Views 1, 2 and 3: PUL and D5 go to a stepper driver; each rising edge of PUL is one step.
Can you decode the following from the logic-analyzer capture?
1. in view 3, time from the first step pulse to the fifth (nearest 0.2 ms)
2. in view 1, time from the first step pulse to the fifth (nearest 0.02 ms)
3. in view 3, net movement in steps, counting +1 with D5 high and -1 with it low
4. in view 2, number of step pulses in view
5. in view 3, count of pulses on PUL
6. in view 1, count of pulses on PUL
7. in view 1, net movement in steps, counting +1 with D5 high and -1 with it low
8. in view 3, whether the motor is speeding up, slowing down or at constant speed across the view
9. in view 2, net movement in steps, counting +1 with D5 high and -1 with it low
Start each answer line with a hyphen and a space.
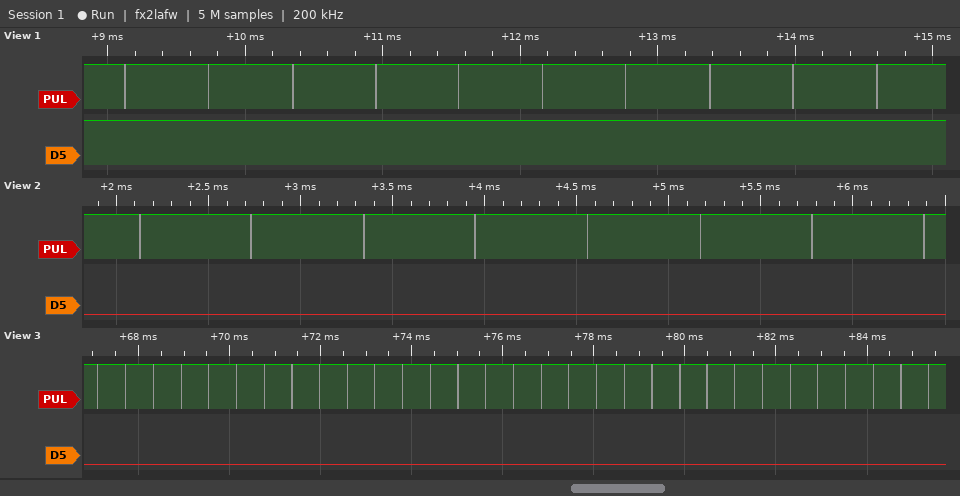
- 2.4 ms
- 2.42 ms
- -31
- 8
- 31
- 10
- +10
- constant speed
- -8
